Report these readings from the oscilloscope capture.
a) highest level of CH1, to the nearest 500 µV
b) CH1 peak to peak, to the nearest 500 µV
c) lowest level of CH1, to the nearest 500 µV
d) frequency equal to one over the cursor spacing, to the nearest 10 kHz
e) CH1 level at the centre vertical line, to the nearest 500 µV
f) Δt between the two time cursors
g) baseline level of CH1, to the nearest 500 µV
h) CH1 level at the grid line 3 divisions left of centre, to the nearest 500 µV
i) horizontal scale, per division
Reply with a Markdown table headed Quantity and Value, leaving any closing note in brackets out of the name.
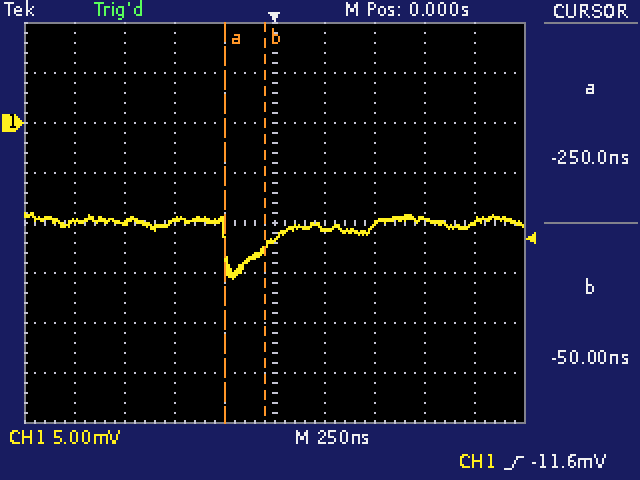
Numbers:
| Quantity | Value |
|---|---|
| highest level of CH1, to the nearest 500 µV | -9.0 mV |
| CH1 peak to peak, to the nearest 500 µV | 6.5 mV |
| lowest level of CH1, to the nearest 500 µV | -15.5 mV |
| frequency equal to one over the cursor spacing, to the nearest 10 kHz | 5.00 MHz |
| CH1 level at the centre vertical line, to the nearest 500 µV | -11.5 mV |
| Δt between the two time cursors | 200 ns |
| baseline level of CH1, to the nearest 500 µV | -10.0 mV |
| CH1 level at the grid line 3 divisions left of centre, to the nearest 500 µV | -10.0 mV |
| horizontal scale, per division | 250 ns |
